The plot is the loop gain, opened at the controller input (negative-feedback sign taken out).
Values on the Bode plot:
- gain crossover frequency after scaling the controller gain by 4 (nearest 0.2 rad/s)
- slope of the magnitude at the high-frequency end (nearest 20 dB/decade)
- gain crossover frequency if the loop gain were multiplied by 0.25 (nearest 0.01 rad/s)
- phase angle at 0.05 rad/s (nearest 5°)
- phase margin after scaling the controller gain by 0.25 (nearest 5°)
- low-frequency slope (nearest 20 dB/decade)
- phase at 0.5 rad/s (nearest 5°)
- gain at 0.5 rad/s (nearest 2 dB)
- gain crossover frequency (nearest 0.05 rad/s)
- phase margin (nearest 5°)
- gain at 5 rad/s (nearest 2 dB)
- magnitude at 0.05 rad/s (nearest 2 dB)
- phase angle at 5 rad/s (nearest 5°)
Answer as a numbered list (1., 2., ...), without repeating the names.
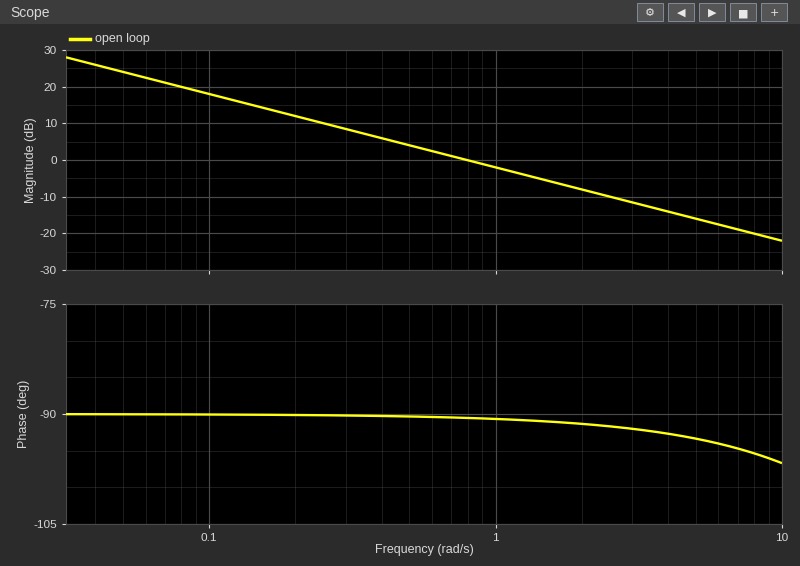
1. 3.2 rad/s
2. -20 dB/decade
3. 0.20 rad/s
4. -90°
5. 90°
6. -20 dB/decade
7. -90°
8. 4 dB
9. 0.80 rad/s
10. 90°
11. -16 dB
12. 24 dB
13. -95°
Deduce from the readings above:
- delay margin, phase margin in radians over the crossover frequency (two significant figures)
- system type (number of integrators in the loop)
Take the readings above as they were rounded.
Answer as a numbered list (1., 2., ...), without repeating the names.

1. 2.0 s
2. 1
